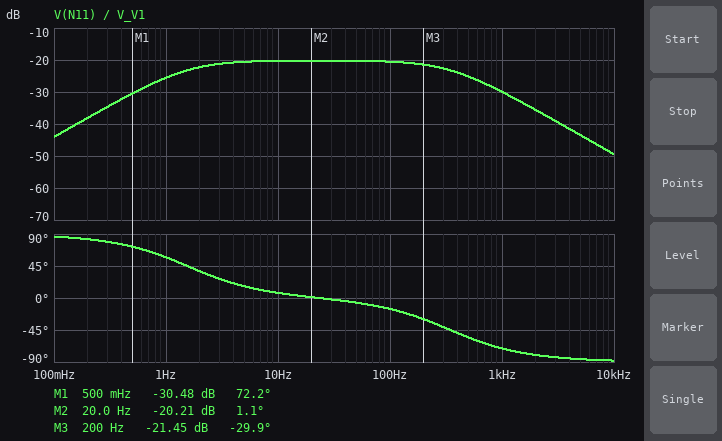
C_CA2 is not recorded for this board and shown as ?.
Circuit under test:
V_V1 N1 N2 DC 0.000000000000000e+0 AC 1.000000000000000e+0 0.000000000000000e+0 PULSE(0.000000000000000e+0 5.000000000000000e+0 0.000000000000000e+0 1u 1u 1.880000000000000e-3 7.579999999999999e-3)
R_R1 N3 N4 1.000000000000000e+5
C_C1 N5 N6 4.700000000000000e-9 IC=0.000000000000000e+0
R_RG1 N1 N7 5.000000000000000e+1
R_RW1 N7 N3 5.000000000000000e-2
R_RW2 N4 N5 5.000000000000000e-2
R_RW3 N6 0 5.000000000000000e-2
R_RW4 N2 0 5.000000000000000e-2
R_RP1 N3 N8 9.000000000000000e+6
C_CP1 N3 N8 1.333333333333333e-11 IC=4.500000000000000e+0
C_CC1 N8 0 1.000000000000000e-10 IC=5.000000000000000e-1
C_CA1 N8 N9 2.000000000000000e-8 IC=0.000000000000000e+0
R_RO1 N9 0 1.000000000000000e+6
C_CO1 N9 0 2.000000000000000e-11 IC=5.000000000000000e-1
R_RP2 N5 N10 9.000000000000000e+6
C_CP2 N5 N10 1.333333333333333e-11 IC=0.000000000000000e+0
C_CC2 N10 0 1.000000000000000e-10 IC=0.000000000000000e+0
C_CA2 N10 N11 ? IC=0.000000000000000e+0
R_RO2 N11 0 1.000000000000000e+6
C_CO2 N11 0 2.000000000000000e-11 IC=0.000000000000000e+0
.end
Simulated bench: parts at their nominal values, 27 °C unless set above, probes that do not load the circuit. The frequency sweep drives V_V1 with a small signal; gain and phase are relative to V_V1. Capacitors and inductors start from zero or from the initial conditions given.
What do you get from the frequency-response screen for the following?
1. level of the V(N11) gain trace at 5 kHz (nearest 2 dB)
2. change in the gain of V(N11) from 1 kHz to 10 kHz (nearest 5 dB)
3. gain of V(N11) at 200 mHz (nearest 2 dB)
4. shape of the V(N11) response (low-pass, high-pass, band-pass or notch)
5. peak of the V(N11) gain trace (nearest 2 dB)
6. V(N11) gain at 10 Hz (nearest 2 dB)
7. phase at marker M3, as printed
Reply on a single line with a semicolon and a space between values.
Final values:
-44 dB; -20 dB; -38 dB; band-pass; -20 dB; -20 dB; -29.9 deg
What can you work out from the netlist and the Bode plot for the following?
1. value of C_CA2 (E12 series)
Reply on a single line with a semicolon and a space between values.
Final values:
10 nF
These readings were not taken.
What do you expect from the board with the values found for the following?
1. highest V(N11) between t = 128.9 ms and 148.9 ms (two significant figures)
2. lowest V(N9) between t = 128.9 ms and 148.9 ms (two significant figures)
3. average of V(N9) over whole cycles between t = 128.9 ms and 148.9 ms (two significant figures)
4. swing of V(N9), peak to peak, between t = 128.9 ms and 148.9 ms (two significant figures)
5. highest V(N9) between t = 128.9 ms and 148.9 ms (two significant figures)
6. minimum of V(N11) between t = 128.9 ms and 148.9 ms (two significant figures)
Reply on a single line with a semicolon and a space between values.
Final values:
390 mV; -68 mV; 62 mV; 510 mV; 440 mV; -94 mV
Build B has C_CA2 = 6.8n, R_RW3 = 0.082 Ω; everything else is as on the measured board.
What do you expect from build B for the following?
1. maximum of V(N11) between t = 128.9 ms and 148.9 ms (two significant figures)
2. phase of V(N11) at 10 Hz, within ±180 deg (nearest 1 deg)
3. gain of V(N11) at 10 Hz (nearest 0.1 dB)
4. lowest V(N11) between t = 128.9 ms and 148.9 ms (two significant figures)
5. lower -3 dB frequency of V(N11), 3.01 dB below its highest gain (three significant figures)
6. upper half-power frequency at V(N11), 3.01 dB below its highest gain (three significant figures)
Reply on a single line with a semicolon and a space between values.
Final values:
370 mV; 11 deg; -20.4 dB; -110 mV; 2.26 Hz; 346 Hz
